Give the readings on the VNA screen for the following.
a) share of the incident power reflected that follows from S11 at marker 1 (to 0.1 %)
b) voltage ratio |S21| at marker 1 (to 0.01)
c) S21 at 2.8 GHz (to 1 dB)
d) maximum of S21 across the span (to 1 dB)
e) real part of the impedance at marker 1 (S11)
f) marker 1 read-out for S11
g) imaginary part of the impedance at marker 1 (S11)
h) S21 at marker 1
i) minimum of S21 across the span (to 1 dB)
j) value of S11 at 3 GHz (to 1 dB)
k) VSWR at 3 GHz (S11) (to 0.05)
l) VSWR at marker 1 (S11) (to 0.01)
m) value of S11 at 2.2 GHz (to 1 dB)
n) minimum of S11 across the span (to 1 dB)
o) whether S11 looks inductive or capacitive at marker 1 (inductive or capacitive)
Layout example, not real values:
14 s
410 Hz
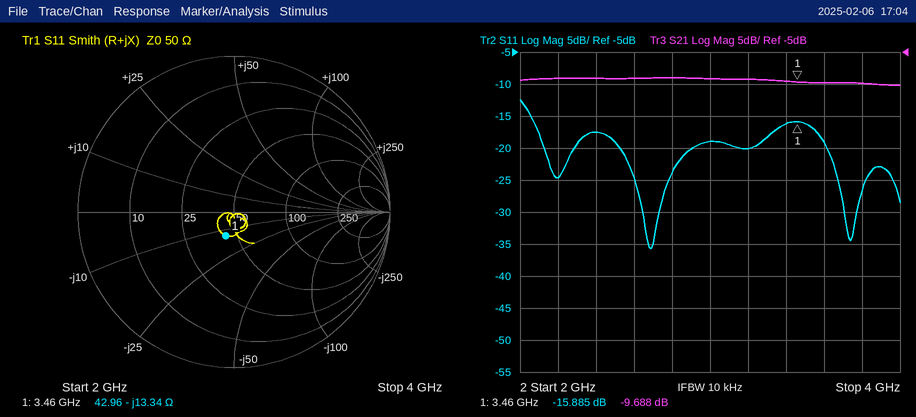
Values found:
2.6 %
0.33
-9 dB
-9 dB
42.96 Ω
-15.885 dB
-13.34 Ω
-9.688 dB
-10 dB
-19 dB
1.25
1.38
-25 dB
-36 dB
capacitive
